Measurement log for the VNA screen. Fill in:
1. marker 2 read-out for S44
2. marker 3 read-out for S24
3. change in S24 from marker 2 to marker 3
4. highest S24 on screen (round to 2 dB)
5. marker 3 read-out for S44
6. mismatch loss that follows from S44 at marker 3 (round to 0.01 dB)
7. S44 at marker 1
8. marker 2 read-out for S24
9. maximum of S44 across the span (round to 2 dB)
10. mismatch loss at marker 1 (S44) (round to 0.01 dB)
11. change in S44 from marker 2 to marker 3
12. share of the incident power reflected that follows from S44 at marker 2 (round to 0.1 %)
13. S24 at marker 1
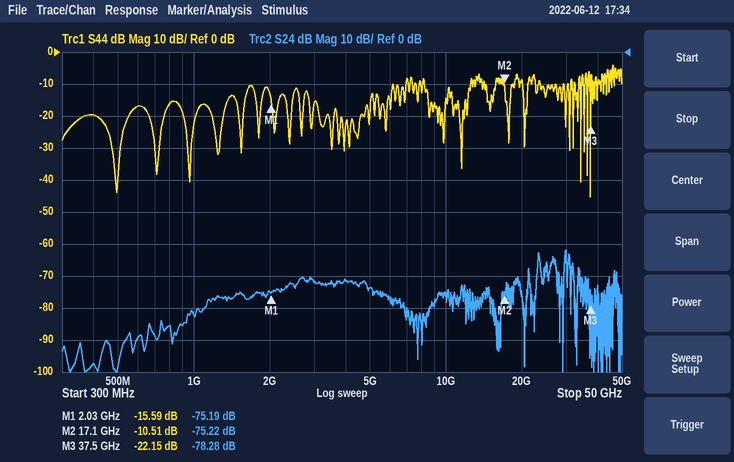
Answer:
-10.51 dB
-78.28 dB
-3.06 dB
-62 dB
-22.15 dB
0.03 dB
-15.59 dB
-75.22 dB
-4 dB
0.12 dB
-11.64 dB
8.9 %
-75.19 dB
